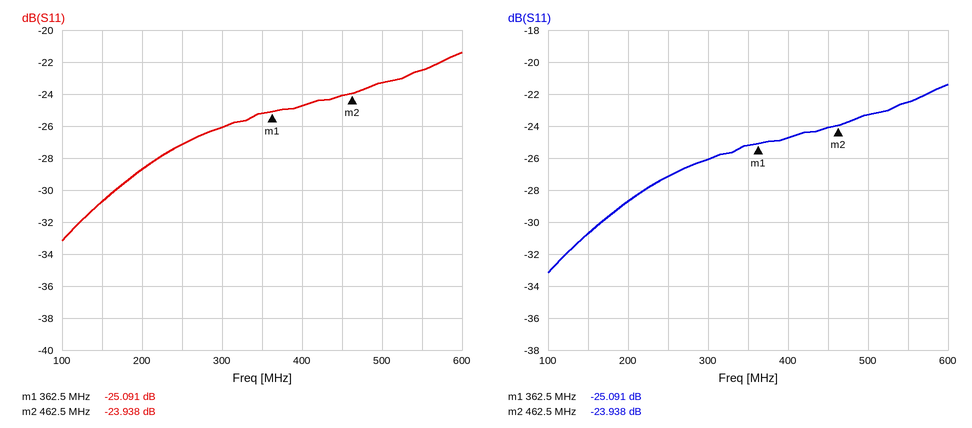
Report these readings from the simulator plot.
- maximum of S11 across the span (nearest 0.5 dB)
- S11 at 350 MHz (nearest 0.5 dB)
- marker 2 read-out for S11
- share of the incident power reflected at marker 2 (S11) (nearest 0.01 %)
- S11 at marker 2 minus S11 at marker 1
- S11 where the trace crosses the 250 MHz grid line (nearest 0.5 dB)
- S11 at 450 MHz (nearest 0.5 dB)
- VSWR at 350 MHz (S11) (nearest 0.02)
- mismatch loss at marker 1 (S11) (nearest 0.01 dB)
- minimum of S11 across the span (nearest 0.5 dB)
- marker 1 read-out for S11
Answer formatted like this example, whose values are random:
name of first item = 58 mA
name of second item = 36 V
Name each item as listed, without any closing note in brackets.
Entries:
maximum of S11 across the span = -21.5 dB
S11 at 350 MHz = -25.0 dB
marker 2 read-out for S11 = -23.938 dB
share of the incident power reflected at marker 2 (S11) = 0.40 %
S11 at marker 2 minus S11 at marker 1 = 1.153 dB
S11 where the trace crosses the 250 MHz grid line = -27.0 dB
S11 at 450 MHz = -24.0 dB
VSWR at 350 MHz (S11) = 1.12
mismatch loss at marker 1 (S11) = 0.01 dB
minimum of S11 across the span = -33.0 dB
marker 1 read-out for S11 = -25.091 dB
